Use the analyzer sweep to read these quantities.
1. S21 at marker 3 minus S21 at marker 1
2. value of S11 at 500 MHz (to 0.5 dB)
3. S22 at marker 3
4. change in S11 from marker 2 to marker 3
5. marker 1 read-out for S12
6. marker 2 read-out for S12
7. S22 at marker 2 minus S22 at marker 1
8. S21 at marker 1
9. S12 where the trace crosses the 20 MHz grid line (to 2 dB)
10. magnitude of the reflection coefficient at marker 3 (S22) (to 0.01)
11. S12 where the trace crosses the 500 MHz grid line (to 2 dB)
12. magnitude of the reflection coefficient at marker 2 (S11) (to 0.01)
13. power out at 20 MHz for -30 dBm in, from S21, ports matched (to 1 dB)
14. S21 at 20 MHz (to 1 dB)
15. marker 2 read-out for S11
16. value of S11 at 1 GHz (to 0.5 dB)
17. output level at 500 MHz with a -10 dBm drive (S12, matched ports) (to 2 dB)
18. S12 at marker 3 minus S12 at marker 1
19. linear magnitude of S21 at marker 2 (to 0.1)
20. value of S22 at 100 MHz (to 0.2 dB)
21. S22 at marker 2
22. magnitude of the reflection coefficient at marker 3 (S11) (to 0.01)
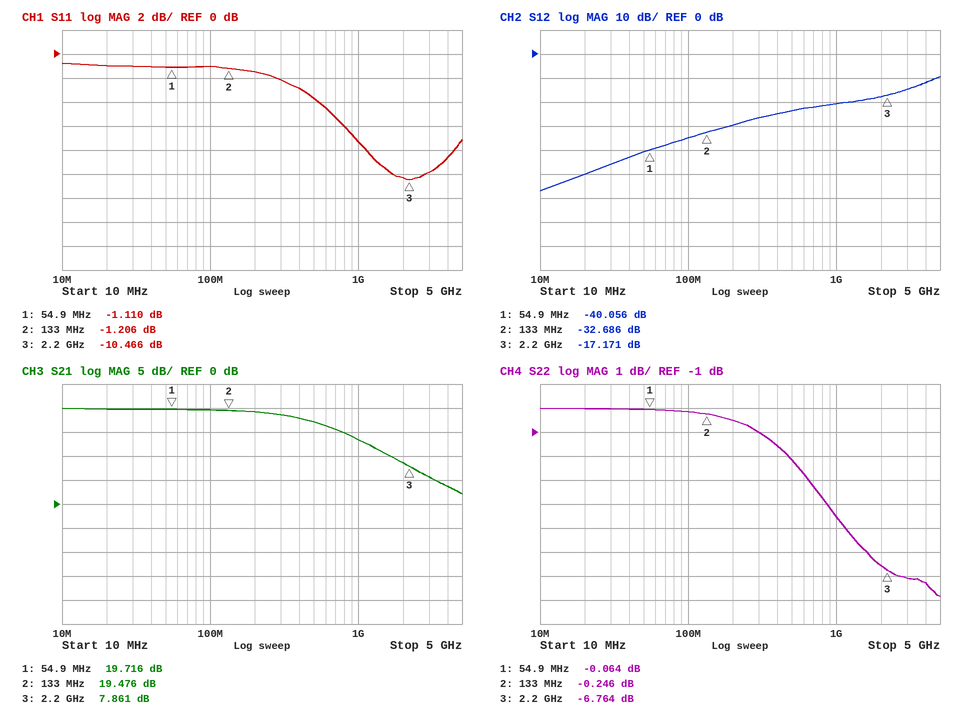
-11.855 dB
-3.5 dB
-6.764 dB
-9.260 dB
-40.056 dB
-32.686 dB
-0.182 dB
19.716 dB
-50 dB
0.46
-24 dB
0.87
-10 dBm
20 dB
-1.206 dB
-7.5 dB
-34 dBm
22.885 dB
9.4
-0.2 dB
-0.246 dB
0.30
